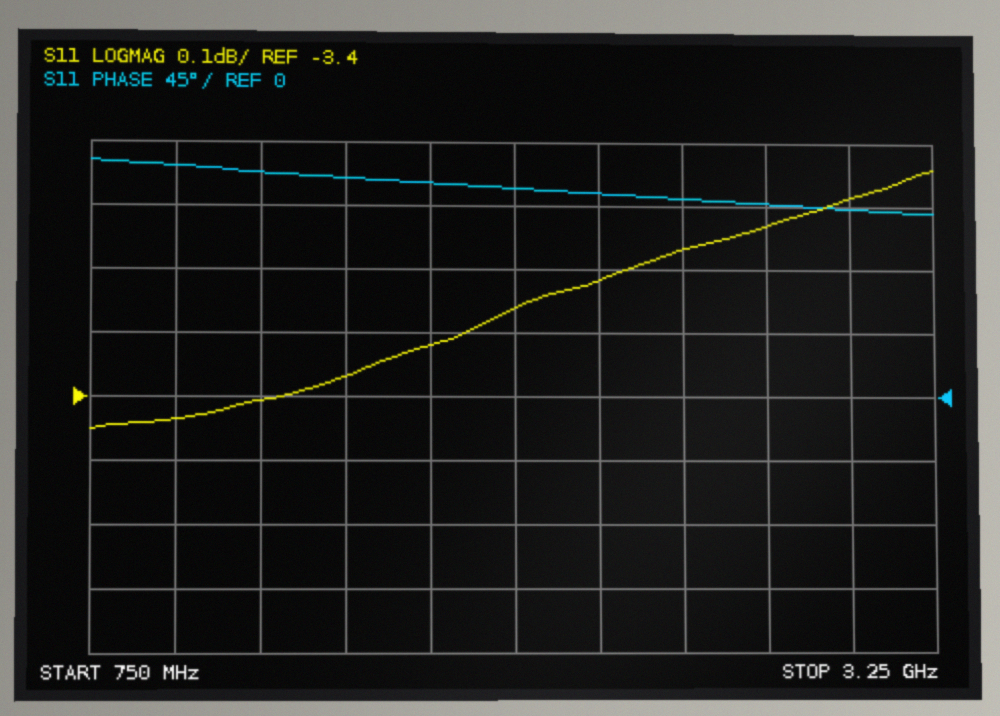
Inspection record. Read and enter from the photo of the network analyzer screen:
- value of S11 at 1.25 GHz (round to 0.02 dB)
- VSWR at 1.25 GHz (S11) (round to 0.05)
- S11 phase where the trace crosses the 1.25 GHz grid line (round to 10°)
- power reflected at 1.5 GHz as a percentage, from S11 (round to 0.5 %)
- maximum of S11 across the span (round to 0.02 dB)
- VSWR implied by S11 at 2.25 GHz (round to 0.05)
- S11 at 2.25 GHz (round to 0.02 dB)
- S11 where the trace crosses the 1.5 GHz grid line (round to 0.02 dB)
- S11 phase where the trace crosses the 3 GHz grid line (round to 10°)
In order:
-3.40 dB
5.15
160°
46.0 %
-3.04 dB
5.45
-3.22 dB
-3.36 dB
130°
